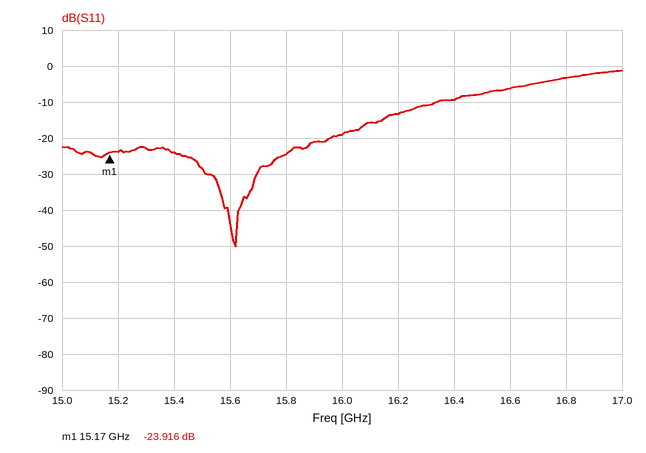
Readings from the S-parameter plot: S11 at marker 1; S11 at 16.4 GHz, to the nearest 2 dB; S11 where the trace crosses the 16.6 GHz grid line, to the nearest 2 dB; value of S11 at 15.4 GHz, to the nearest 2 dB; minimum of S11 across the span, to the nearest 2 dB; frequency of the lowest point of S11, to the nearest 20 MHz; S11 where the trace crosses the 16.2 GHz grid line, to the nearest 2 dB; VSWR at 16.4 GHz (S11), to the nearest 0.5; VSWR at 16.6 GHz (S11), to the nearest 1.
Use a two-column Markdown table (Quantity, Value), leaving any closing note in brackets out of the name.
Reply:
| Quantity | Value |
|---|---|
| S11 at marker 1 | -23.916 dB |
| S11 at 16.4 GHz, to the nearest 2 dB | -10 dB |
| S11 where the trace crosses the 16.6 GHz grid line, to the nearest 2 dB | -6 dB |
| value of S11 at 15.4 GHz, to the nearest 2 dB | -24 dB |
| minimum of S11 across the span, to the nearest 2 dB | -50 dB |
| frequency of the lowest point of S11, to the nearest 20 MHz | 15.62 GHz |
| S11 where the trace crosses the 16.2 GHz grid line, to the nearest 2 dB | -14 dB |
| VSWR at 16.4 GHz (S11), to the nearest 0.5 | 2.0 |
| VSWR at 16.6 GHz (S11), to the nearest 1 | 3 |
